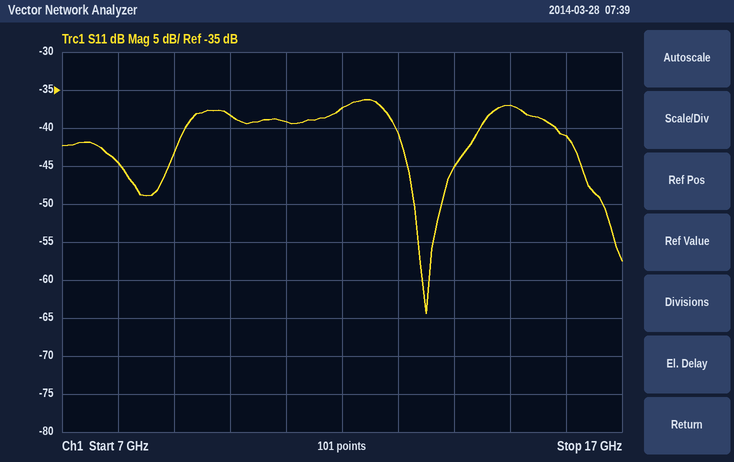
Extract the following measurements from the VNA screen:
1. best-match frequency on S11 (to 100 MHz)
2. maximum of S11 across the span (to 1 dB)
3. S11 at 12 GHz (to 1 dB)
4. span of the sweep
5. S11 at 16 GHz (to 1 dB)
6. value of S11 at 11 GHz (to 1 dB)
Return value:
13.5 GHz
-36 dB
-37 dB
10 GHz
-41 dB
-39 dB
